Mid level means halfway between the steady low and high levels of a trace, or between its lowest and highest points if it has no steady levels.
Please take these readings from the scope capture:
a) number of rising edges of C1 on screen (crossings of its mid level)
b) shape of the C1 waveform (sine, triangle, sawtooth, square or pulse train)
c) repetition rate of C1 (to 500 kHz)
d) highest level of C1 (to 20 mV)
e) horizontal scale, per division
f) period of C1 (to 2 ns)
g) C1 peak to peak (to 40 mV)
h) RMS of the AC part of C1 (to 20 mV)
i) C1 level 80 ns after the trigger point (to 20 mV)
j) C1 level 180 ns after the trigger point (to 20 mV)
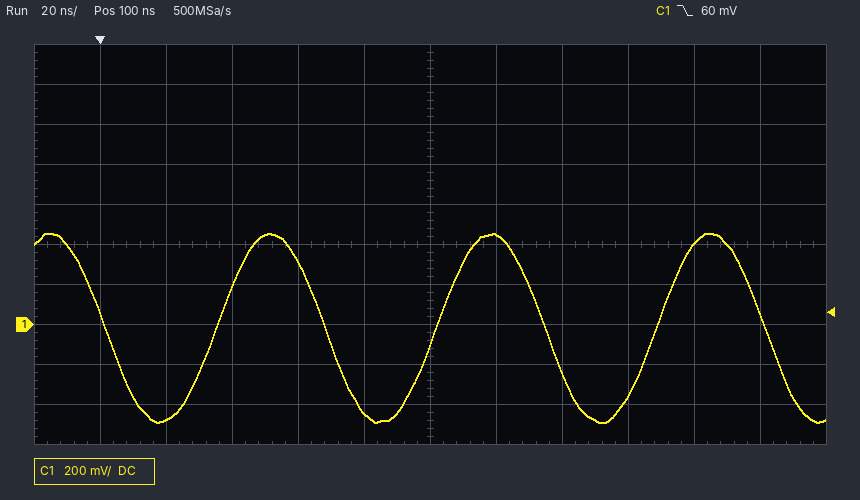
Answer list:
3
sine
15.0 MHz
460 mV
20 ns
66 ns
960 mV
340 mV
-440 mV
400 mV
